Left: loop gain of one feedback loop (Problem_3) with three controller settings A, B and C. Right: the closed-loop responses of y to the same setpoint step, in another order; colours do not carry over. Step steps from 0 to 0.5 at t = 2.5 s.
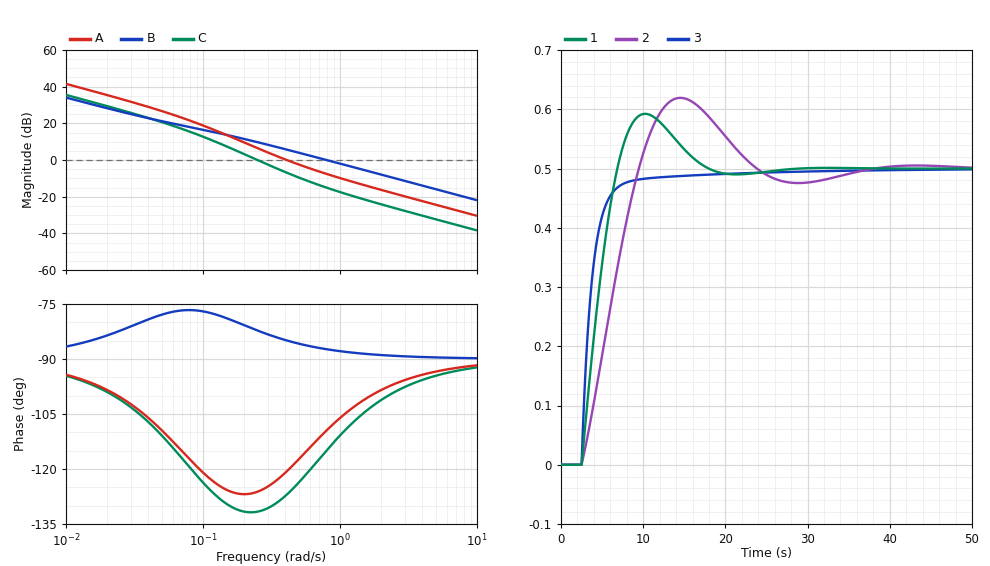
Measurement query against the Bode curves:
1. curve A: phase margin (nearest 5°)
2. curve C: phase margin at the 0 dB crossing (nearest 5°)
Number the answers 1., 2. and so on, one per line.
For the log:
1. 60°
2. 50°
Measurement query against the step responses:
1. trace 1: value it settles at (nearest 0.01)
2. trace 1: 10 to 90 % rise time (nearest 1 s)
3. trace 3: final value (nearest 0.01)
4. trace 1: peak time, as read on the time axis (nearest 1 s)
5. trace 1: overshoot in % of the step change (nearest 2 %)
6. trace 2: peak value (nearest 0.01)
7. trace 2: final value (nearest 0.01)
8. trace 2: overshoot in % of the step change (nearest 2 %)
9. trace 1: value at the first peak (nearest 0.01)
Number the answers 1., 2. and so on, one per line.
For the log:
1. 0.50
2. 3 s
3. 0.50
4. 10 s
5. 18 %
6. 0.62
7. 0.50
8. 24 %
9. 0.59
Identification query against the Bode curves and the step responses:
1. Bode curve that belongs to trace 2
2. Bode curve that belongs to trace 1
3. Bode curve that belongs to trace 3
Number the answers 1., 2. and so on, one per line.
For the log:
1. C
2. A
3. B
